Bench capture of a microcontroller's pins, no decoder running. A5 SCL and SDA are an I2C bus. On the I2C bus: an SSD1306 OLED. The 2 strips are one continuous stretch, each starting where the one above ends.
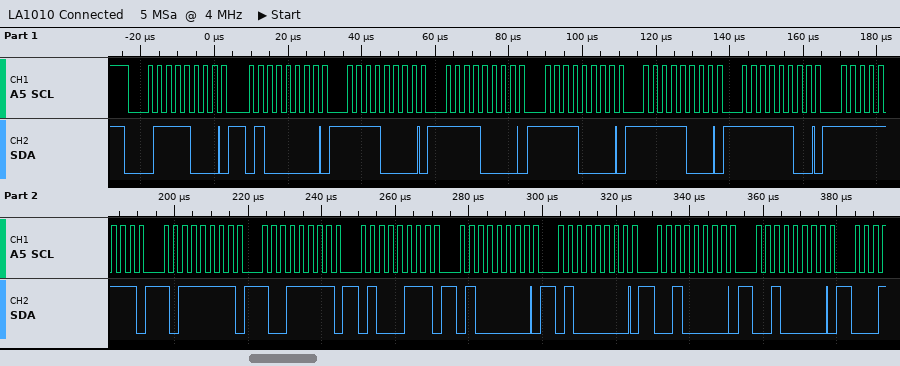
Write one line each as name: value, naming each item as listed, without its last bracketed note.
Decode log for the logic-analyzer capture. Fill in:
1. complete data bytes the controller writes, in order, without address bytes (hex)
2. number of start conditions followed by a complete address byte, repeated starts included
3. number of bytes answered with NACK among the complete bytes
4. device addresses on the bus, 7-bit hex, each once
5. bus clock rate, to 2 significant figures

complete data bytes the controller writes, in order, without address bytes: 40 F0 F0 F0 F8 FC FF BF 9F 47 40 40 20 20
number of start conditions followed by a complete address byte, repeated starts included: 1
number of bytes answered with NACK among the complete bytes: 0
device addresses on the bus, 7-bit hex, each once: 0x3C
bus clock rate, to 2 significant figures: 400 kHz
